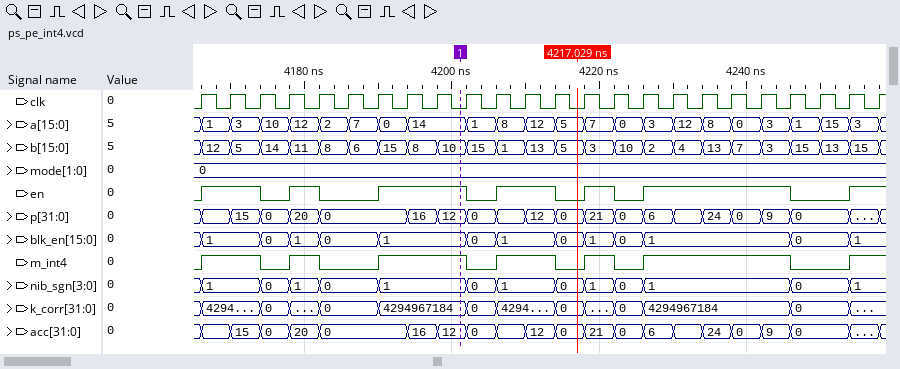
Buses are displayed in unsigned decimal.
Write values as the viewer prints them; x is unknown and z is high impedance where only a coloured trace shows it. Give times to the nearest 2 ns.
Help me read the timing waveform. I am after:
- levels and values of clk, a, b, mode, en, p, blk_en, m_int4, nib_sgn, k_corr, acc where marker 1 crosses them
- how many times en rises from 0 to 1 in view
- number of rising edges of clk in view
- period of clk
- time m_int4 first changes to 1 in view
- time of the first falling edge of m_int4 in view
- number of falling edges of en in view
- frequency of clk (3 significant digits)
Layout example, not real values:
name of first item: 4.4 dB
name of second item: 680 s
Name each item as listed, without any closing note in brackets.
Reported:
levels and values of clk, a, b, mode, en, p, blk_en, m_int4, nib_sgn, k_corr, acc where marker 1 crosses them: clk=0, a=14, b=10, mode=0, en=1, p=12, blk_en=1, m_int4=1, nib_sgn=1, k_corr=4294967184, acc=12
how many times en rises from 0 to 1 in view: 7
number of rising edges of clk in view: 24
period of clk: 4 ns
time m_int4 first changes to 1 in view: 4166 ns
time of the first falling edge of m_int4 in view: 4174 ns
number of falling edges of en in view: 6
frequency of clk: 250 MHz
